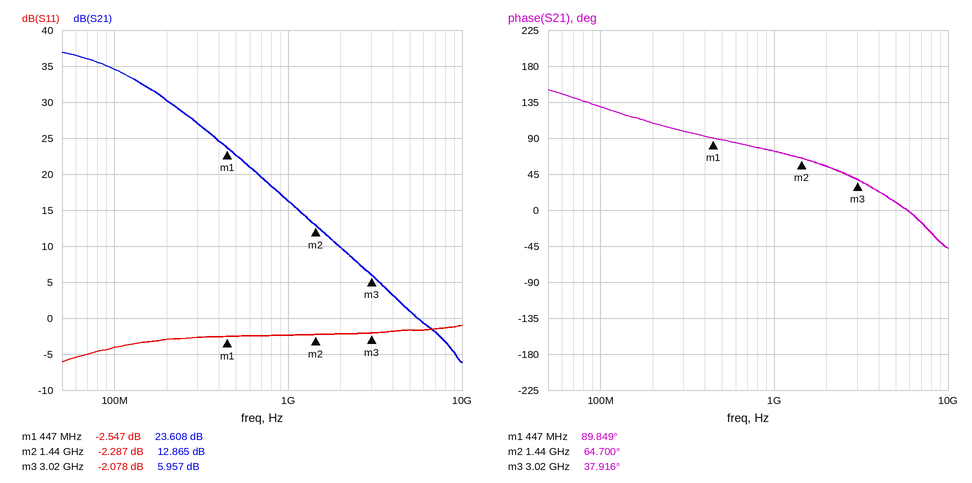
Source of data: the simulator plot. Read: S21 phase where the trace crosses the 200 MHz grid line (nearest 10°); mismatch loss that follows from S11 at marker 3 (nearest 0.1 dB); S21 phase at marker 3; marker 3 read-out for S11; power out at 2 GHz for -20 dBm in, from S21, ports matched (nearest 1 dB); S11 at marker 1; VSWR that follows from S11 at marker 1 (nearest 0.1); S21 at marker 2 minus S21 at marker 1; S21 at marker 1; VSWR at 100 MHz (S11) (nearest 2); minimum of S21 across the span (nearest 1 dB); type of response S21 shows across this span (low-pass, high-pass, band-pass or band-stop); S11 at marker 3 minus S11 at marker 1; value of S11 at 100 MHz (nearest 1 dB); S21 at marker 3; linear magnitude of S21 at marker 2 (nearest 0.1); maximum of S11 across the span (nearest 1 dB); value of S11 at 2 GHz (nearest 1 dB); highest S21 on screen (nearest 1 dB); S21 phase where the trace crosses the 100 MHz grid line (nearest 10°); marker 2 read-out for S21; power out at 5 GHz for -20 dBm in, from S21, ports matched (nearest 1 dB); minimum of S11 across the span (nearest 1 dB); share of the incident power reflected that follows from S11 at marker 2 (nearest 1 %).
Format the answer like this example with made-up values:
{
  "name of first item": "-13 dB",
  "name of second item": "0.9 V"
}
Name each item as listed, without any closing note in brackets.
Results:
{
  "S21 phase where the trace crosses the 200 MHz grid line": "110°",
  "mismatch loss that follows from S11 at marker 3": "4.2 dB",
  "S21 phase at marker 3": "37.916°",
  "marker 3 read-out for S11": "-2.078 dB",
  "power out at 2 GHz for -20 dBm in, from S21, ports matched": "-10 dBm",
  "S11 at marker 1": "-2.547 dB",
  "VSWR that follows from S11 at marker 1": "6.9",
  "S21 at marker 2 minus S21 at marker 1": "-10.743 dB",
  "S21 at marker 1": "23.608 dB",
  "VSWR at 100 MHz (S11)": "4",
  "minimum of S21 across the span": "-6 dB",
  "type of response S21 shows across this span": "low-pass",
  "S11 at marker 3 minus S11 at marker 1": "0.469 dB",
  "value of S11 at 100 MHz": "-4 dB",
  "S21 at marker 3": "5.957 dB",
  "linear magnitude of S21 at marker 2": "4.4",
  "maximum of S11 across the span": "-1 dB",
  "value of S11 at 2 GHz": "-2 dB",
  "highest S21 on screen": "37 dB",
  "S21 phase where the trace crosses the 100 MHz grid line": "130°",
  "marker 2 read-out for S21": "12.865 dB",
  "power out at 5 GHz for -20 dBm in, from S21, ports matched": "-19 dBm",
  "minimum of S11 across the span": "-6 dB",
  "share of the incident power reflected that follows from S11 at marker 2": "59 %"
}
